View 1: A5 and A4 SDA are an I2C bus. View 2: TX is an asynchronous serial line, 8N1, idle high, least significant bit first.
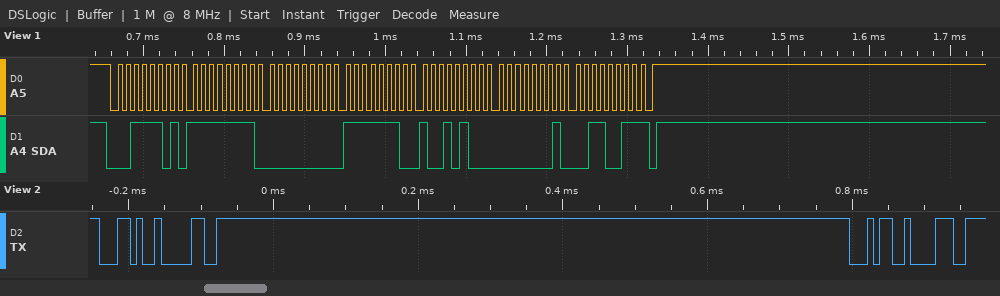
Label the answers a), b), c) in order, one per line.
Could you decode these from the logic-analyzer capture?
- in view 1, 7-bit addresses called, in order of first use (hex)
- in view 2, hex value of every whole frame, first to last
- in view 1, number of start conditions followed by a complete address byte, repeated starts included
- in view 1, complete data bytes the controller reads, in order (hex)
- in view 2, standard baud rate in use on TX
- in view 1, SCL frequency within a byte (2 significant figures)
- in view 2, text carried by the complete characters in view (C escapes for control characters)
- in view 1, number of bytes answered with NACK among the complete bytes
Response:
a) 0x1E
b) 2C 30 34 38
c) 1
d) FF 00 FE 94 01 33
e) 115200 baud
f) 100 kHz
g) ",048"
h) 1
